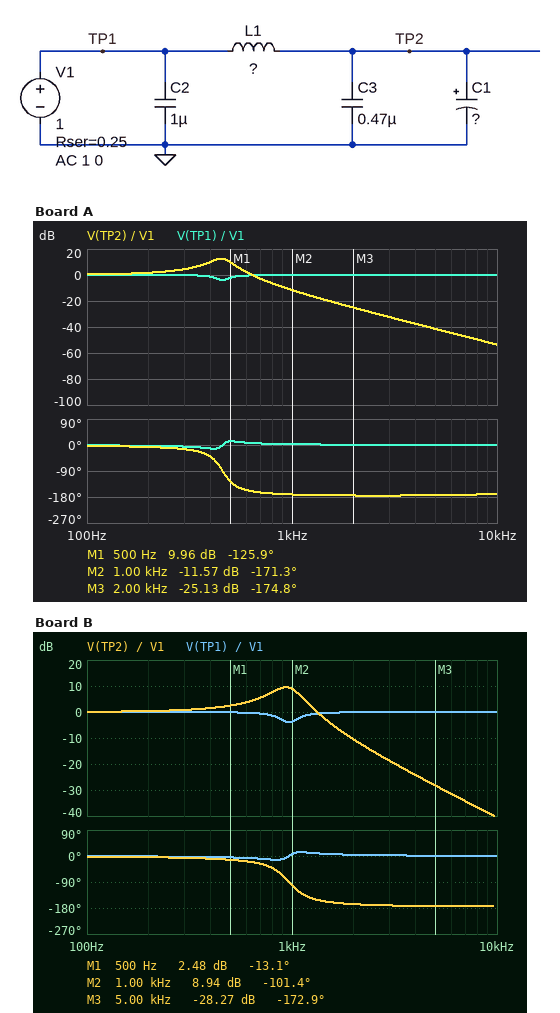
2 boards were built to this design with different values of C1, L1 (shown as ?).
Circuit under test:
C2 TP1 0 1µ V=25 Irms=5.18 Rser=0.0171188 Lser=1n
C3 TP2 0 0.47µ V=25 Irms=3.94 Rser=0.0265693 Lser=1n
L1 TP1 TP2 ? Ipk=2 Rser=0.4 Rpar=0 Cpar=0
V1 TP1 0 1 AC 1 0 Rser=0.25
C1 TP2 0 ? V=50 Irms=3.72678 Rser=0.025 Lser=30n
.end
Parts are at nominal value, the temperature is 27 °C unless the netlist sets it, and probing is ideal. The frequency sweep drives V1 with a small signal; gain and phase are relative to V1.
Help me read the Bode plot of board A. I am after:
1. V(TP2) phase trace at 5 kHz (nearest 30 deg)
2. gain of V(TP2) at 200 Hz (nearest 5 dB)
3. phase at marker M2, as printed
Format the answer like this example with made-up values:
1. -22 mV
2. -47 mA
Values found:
1. -180 deg
2. 0 dB
3. -171.3 deg
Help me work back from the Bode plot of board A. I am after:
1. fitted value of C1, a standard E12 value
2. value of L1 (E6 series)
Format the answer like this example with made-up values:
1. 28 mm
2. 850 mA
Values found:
1. 120 µF
2. 1 mH
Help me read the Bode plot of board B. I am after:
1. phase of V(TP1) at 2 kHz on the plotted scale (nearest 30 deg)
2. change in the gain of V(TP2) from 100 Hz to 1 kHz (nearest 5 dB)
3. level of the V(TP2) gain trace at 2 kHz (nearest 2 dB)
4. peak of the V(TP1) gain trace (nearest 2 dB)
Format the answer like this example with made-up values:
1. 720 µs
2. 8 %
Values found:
1. 0 deg
2. 10 dB
3. -10 dB
4. 0 dB
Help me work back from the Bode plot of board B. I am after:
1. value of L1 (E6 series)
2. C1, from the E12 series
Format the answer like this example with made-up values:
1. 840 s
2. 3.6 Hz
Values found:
1. 330 µH
2. 82 µF
